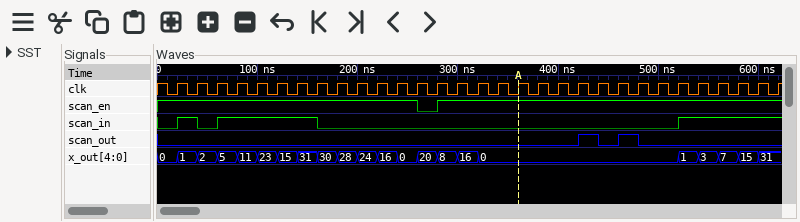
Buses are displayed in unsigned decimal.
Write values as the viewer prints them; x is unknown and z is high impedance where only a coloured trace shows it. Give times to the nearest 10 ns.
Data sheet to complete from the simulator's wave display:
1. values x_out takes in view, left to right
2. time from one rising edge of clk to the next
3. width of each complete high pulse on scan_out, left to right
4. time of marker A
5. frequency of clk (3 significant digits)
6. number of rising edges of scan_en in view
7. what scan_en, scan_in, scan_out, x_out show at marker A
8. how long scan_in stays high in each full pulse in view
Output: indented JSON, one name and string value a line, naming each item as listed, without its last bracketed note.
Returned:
{
  "values x_out takes in view, left to right": "0, 1, 2, 5, 11, 23, 15, 31, 30, 28, 24, 16, 0, 20, 8, 16, 0, 1, 3, 7, 15, 31",
  "time from one rising edge of clk to the next": "20 ns",
  "width of each complete high pulse on scan_out, left to right": "20 ns, 20 ns",
  "time of marker A": "360 ns",
  "frequency of clk": "50.0 MHz",
  "number of rising edges of scan_en in view": "1",
  "what scan_en, scan_in, scan_out, x_out show at marker A": "scan_en=1, scan_in=0, scan_out=0, x_out=0",
  "how long scan_in stays high in each full pulse in view": "20 ns, 100 ns"
}
